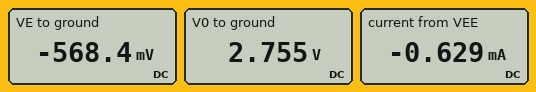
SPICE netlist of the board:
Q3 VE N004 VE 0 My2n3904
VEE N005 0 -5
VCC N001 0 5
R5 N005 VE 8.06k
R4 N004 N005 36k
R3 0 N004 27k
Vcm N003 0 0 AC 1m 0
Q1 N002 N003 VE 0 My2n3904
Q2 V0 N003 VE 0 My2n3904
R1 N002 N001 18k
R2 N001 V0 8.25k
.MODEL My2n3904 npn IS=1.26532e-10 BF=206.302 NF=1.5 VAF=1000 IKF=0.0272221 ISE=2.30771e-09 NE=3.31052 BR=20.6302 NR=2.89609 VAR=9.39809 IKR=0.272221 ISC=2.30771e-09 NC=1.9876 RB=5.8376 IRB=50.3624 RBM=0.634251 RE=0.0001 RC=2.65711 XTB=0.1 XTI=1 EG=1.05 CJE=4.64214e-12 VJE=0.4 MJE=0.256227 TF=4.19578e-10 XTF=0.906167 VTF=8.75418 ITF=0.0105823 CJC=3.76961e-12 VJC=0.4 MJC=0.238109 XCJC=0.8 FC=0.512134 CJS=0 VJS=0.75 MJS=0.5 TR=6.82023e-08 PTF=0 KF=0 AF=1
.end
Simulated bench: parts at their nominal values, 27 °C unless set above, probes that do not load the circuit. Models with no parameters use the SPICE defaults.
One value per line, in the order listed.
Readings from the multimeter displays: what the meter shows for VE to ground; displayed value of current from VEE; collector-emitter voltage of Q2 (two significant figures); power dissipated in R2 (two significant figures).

-568.4 mV
-0.629 mA
3.3 V
610 µW
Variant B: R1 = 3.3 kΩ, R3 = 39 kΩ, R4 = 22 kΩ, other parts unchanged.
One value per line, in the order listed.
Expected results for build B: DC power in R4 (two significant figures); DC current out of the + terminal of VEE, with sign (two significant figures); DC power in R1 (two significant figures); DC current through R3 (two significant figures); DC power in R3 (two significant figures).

150 µW
-630 µA
240 µW
82 µA
260 µW
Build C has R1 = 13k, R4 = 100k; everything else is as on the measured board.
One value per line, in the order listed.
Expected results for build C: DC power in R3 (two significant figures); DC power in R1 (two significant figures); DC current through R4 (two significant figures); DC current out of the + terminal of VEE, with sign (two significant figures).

42 µW
960 µW
39 µA
-590 µA
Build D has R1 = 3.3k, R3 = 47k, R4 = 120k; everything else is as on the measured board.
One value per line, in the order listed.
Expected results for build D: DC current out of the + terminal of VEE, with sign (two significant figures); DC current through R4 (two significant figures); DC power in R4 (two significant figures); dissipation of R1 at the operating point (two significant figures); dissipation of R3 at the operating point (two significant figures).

-580 µA
30 µA
110 µW
240 µW
42 µW
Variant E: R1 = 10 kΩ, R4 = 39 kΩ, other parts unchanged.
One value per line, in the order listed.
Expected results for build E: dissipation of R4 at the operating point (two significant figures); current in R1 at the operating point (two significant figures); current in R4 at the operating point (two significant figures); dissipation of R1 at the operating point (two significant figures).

220 µW
270 µA
76 µA
740 µW
